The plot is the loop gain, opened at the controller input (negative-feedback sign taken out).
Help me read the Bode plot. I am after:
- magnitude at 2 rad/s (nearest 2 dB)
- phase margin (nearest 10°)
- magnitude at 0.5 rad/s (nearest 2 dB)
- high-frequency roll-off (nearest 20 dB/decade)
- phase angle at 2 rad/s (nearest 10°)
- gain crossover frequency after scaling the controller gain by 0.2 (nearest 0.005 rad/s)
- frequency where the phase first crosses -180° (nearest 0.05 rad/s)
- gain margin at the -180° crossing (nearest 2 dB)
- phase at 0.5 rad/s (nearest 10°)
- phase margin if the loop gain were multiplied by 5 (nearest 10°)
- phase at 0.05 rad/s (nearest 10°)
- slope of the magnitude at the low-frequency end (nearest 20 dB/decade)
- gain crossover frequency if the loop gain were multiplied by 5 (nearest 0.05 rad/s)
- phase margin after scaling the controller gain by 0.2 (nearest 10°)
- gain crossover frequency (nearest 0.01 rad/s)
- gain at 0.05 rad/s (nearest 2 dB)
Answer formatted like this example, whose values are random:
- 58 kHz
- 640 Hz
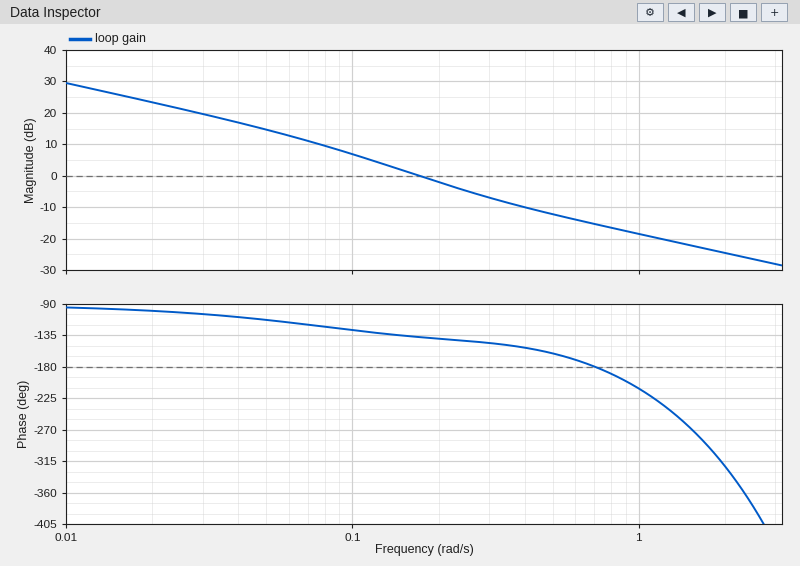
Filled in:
- -24 dB
- 40°
- -12 dB
- -20 dB/decade
- -320°
- 0.055 rad/s
- 0.70 rad/s
- 16 dB
- -160°
- 10°
- -110°
- -20 dB/decade
- 0.60 rad/s
- 70°
- 0.17 rad/s
- 14 dB
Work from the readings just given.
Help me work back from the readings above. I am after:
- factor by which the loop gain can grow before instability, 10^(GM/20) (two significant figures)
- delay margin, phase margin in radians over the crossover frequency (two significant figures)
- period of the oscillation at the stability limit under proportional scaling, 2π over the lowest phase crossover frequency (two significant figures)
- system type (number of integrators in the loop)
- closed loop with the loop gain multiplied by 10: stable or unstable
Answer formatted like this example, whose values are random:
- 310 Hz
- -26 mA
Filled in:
- 6.3
- 4.1 s
- 9.0 s
- 1
- unstable
